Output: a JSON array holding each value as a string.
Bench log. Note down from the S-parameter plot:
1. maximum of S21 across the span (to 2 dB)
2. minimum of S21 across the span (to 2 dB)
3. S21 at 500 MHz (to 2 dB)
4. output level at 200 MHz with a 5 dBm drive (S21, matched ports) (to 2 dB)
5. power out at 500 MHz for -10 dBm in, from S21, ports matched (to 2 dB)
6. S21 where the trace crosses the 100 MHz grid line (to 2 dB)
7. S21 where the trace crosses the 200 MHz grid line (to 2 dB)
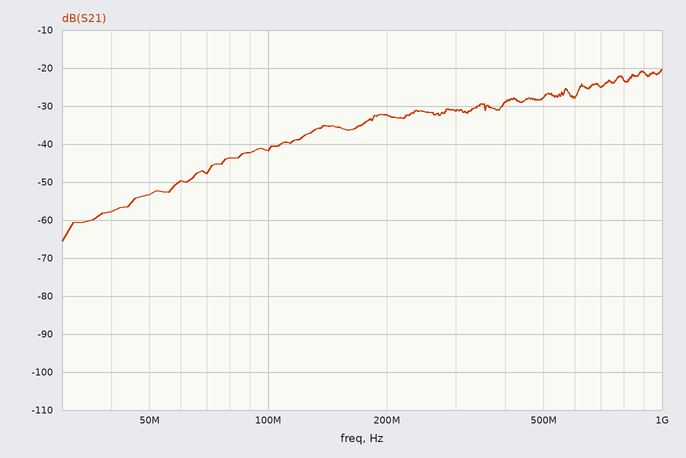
["-20 dB", "-66 dB", "-28 dB", "-28 dBm", "-38 dBm", "-42 dB", "-32 dB"]
